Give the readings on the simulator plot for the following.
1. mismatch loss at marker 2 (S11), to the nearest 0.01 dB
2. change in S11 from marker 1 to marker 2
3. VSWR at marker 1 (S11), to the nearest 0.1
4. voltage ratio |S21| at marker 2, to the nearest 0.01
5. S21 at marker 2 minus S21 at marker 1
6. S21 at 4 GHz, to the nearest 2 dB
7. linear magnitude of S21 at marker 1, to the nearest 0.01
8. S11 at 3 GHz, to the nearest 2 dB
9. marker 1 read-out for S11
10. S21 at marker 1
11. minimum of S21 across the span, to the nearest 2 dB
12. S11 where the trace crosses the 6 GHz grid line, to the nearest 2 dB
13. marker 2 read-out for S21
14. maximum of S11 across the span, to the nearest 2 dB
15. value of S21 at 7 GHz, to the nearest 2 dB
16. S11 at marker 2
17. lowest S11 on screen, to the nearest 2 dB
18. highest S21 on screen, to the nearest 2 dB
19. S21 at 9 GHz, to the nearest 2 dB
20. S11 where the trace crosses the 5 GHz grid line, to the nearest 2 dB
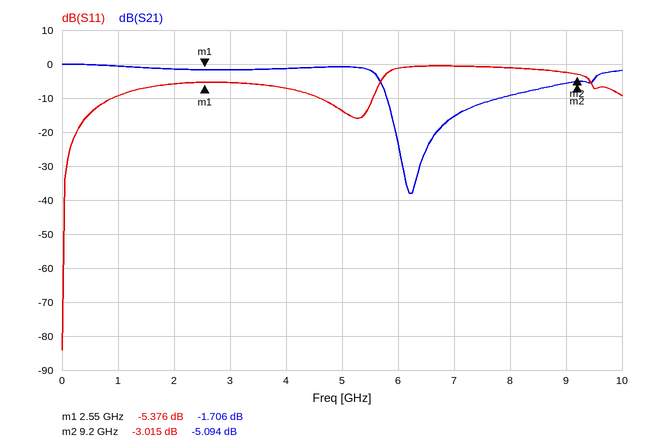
3.01 dB
2.361 dB
3.3
0.56
-3.388 dB
-2 dB
0.82
-6 dB
-5.376 dB
-1.706 dB
-38 dB
-2 dB
-5.094 dB
0 dB
-16 dB
-3.015 dB
-84 dB
0 dB
-6 dB
-14 dB
